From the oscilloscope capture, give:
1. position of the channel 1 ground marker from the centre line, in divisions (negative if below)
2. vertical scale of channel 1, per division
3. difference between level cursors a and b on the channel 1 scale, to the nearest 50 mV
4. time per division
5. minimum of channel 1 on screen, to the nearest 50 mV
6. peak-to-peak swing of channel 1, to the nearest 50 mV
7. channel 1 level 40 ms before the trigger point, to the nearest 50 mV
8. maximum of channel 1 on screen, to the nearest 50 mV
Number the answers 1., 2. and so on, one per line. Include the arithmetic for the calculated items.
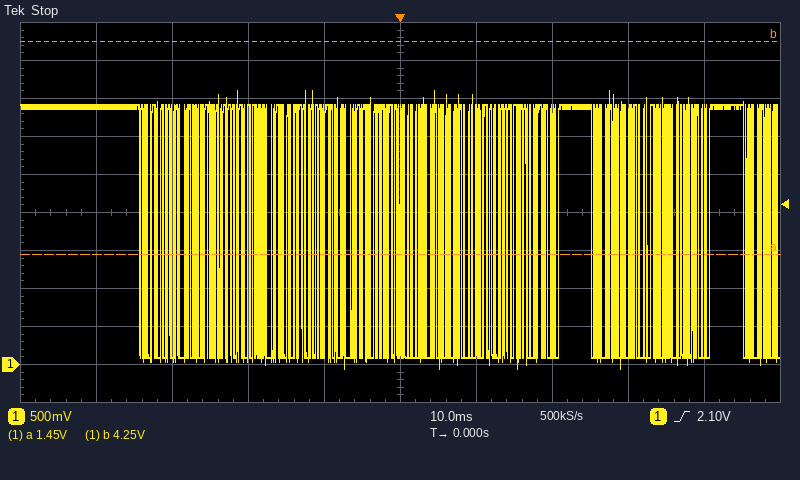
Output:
1. -4.0 div
2. 500 mV
3. 2.80 V
4. 10 ms
5. -50 mV
6. 3.60 V − (-50 mV) = 3.65 V
7. 3.40 V
8. 3.60 V
